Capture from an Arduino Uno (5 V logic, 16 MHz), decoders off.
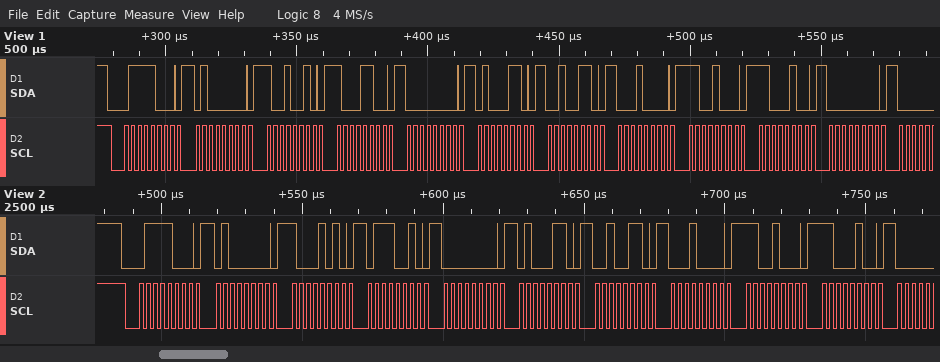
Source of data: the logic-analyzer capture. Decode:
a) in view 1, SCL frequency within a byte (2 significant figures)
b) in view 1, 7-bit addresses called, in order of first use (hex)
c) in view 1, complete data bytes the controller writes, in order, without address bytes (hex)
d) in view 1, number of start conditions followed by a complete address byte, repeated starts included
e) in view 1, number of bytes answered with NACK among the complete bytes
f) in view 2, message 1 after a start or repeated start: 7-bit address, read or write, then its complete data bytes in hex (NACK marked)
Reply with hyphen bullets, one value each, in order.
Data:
- 400 kHz
- 0x3C
- 40 92 8C 00 46 26 10 C8 C4 00
- 1
- 0
- 0x3C write: 40 8A 72 00 46 26 10 C8 C4
